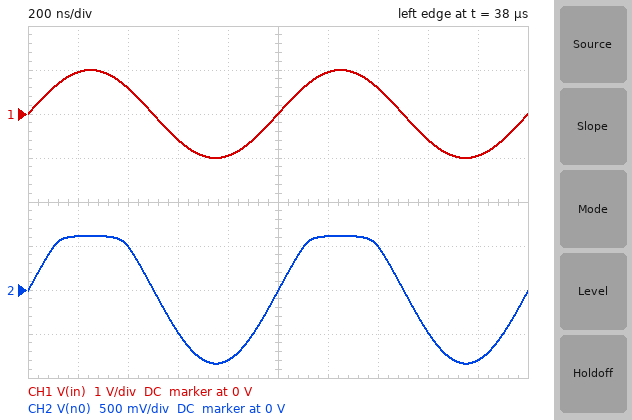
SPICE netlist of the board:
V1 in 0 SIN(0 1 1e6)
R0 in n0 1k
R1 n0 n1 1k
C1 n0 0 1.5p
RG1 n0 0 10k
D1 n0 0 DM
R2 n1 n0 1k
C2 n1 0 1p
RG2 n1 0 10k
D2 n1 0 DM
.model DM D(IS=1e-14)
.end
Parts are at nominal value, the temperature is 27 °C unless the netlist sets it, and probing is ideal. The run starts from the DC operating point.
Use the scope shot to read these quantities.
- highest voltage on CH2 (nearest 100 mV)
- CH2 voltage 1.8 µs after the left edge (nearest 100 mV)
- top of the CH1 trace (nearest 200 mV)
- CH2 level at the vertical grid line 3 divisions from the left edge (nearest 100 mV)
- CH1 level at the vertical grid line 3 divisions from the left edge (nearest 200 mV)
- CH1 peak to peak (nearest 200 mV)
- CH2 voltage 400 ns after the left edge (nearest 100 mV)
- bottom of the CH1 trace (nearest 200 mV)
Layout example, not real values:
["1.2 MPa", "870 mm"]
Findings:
["600 mV", "-800 mV", "1.0 V", "-500 mV", "-600 mV", "2.0 V", "500 mV", "-1.0 V"]
